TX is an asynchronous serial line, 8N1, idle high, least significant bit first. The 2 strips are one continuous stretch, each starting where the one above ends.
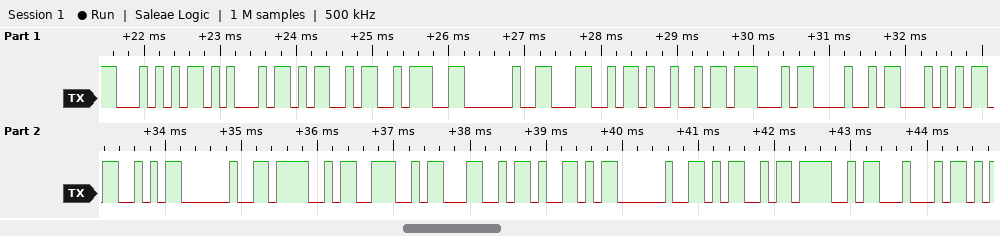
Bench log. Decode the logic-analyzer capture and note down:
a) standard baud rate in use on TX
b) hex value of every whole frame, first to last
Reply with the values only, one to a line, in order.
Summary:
9600 baud
54 45 4D 3A 20 4C 49 47 48 54 53 20 4F 4E 4C 59 20 4D 4F 44
